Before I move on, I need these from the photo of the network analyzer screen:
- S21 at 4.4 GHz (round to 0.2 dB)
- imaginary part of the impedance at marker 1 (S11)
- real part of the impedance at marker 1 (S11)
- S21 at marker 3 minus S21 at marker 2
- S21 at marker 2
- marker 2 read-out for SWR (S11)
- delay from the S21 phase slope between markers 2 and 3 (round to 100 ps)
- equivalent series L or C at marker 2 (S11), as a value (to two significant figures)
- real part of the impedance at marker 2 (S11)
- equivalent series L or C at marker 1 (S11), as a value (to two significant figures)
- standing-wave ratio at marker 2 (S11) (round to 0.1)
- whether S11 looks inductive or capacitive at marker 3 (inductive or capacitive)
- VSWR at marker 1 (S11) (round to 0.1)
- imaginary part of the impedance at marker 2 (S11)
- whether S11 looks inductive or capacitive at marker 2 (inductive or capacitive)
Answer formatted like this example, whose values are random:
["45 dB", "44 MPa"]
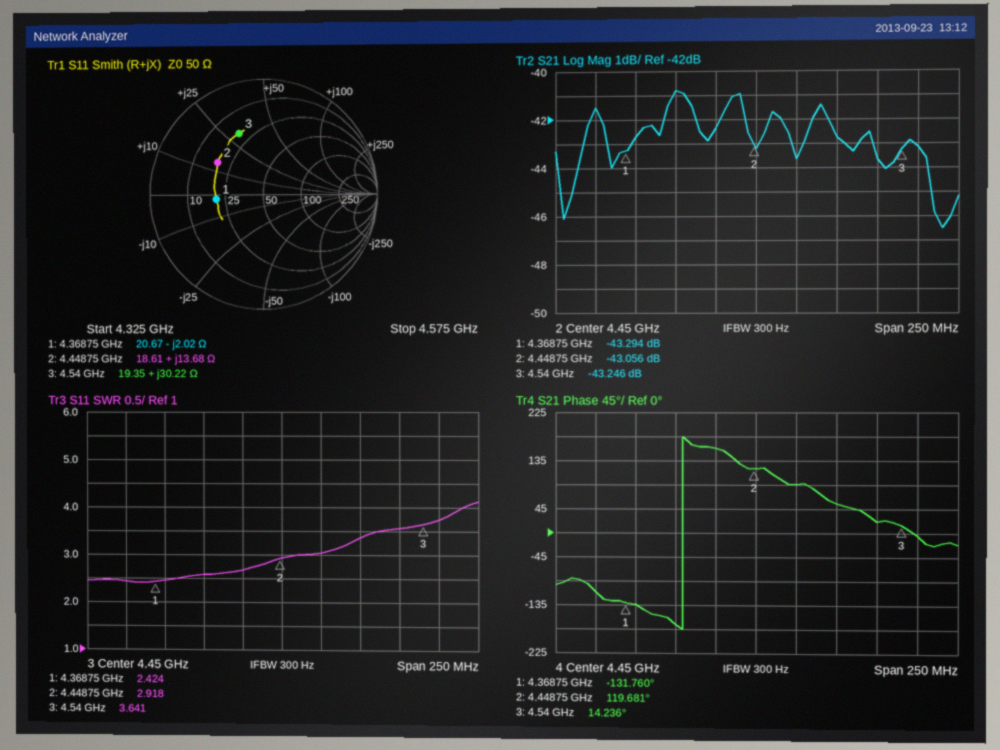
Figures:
["-40.8 dB", "-2.02 Ω", "20.67 Ω", "-0.190 dB", "-43.056 dB", "2.918", "3.2 ns", "490 pH", "18.61 Ω", "18 pF", "2.9", "inductive", "2.4", "+13.68 Ω", "inductive"]
